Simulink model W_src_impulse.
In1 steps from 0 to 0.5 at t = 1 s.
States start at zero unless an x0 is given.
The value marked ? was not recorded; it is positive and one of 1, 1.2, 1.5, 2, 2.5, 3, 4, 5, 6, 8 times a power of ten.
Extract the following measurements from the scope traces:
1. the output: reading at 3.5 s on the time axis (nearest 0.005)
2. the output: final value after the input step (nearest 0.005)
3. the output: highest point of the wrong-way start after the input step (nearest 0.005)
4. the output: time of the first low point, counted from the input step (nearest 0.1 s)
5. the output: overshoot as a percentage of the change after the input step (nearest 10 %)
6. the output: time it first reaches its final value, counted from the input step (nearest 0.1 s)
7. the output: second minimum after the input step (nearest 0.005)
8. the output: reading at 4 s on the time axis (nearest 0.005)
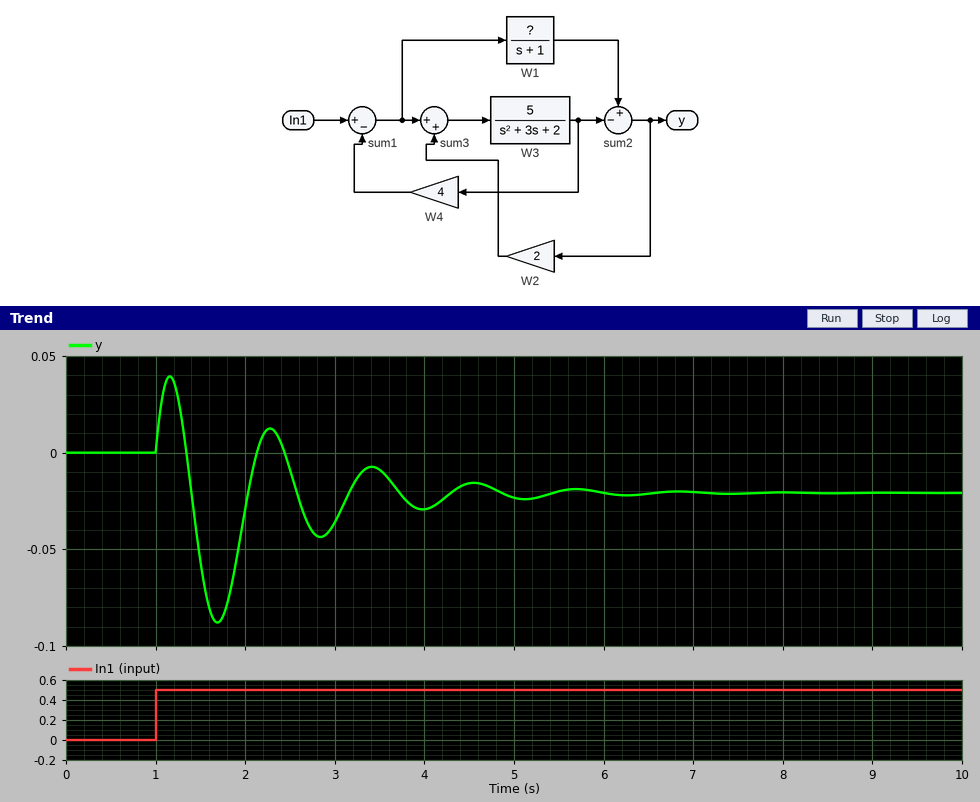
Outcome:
-0.010
-0.020
0.040
0.7 s
320 %
0.4 s
-0.045
-0.030
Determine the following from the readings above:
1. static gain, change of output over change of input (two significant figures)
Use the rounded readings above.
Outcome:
-0.040
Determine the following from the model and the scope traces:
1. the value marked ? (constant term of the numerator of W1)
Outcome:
1
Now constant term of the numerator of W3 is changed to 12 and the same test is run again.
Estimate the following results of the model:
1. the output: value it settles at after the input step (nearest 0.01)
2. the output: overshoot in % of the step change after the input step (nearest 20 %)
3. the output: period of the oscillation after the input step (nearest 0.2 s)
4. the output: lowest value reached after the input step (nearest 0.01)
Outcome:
-0.03
280 %
0.8 s
-0.11
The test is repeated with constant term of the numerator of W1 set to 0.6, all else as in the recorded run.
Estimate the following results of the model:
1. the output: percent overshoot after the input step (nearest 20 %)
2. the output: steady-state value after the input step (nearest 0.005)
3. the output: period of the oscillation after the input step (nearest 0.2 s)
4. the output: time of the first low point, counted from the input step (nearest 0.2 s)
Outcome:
160 %
-0.035
1.2 s
0.6 s
